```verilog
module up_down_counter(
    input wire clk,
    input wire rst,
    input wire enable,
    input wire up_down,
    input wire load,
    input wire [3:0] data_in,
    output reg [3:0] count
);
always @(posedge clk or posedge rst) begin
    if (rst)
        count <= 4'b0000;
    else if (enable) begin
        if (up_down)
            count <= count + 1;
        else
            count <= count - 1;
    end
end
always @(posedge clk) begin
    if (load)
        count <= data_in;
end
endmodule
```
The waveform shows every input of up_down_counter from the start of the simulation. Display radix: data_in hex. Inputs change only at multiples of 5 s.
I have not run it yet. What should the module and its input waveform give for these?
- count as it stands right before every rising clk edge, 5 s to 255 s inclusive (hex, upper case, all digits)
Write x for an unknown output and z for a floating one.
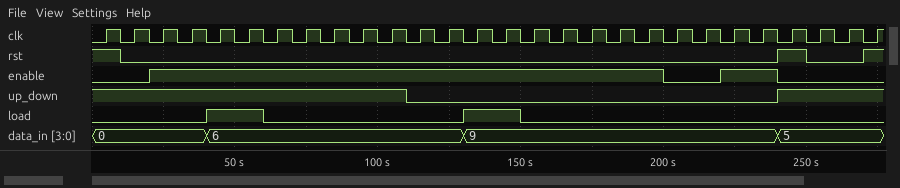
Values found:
0, 0, 0, 1, 2, 6, 6, 7, 8, 9, A, B, A, 9, 9, 9, 8, 7, 6, 5, 4, 4, 4, 3, 0, 0
